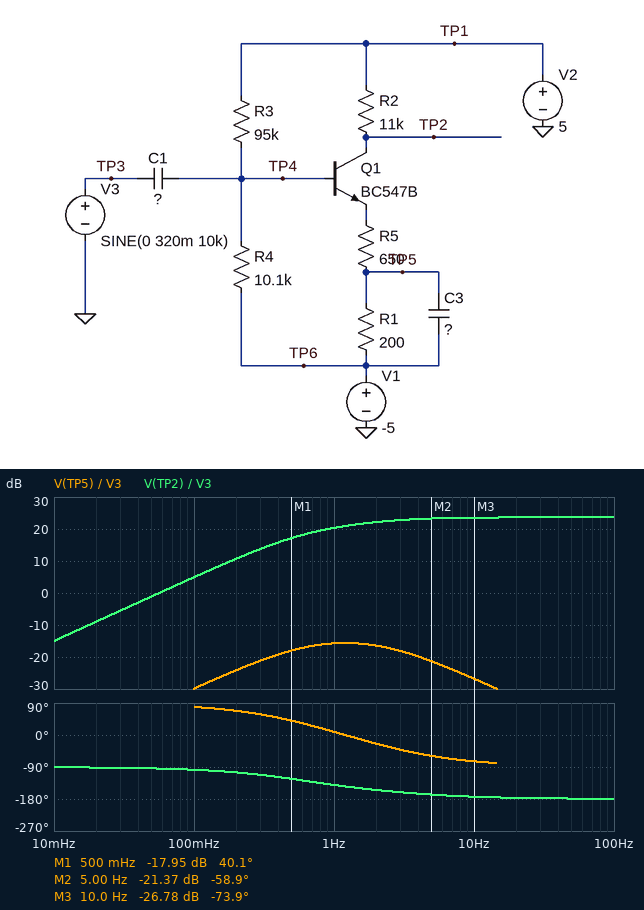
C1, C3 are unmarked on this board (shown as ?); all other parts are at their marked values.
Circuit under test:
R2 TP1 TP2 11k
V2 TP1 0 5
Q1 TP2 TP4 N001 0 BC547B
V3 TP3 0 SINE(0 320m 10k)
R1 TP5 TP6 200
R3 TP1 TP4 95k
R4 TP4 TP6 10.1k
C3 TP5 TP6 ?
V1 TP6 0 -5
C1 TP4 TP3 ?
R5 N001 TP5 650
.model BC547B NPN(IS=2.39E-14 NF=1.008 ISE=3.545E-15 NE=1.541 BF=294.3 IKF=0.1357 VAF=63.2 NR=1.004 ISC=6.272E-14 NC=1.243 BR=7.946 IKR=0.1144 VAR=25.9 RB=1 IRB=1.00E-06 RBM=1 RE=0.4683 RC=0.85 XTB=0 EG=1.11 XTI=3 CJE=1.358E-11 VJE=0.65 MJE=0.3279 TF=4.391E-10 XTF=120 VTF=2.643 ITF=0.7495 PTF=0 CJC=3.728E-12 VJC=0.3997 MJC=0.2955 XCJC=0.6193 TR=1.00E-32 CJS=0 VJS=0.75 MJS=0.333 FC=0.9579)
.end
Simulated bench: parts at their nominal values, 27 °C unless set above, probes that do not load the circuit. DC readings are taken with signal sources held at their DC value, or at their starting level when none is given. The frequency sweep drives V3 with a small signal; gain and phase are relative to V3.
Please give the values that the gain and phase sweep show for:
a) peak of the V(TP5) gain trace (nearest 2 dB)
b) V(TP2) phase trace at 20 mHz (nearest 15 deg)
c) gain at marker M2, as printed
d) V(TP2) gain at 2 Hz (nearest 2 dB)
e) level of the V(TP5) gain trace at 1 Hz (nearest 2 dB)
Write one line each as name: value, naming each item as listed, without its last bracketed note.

peak of the V(TP5) gain trace: -16 dB
V(TP2) phase trace at 20 mHz: -90 deg
gain at marker M2, as printed: -21.37 dB
V(TP2) gain at 2 Hz: 22 dB
level of the V(TP5) gain trace at 1 Hz: -16 dB
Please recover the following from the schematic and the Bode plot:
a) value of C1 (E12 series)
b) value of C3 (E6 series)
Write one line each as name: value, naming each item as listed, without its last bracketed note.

value of C1: 27 µF
value of C3: 470 µF
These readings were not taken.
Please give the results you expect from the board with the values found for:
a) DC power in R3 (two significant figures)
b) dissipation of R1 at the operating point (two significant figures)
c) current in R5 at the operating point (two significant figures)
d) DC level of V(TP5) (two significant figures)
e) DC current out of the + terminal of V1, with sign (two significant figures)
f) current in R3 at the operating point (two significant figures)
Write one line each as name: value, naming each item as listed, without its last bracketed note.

DC power in R3: 860 µW
dissipation of R1 at the operating point: 31 µW
current in R5 at the operating point: 400 µA
DC level of V(TP5): -4.9 V
DC current out of the + terminal of V1, with sign: -490 µA
current in R3 at the operating point: 95 µA
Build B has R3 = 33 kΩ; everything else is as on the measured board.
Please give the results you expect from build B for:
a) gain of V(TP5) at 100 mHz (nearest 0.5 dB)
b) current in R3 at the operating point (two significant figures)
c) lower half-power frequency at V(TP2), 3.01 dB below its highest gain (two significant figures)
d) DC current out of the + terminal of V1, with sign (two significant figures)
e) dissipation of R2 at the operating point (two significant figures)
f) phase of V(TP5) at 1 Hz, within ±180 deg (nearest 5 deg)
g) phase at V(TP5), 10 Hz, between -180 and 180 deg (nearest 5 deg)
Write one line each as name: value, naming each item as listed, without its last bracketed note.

gain of V(TP5) at 100 mHz: -51.0 dB
current in R3 at the operating point: 260 µA
lower half-power frequency at V(TP2), 3.01 dB below its highest gain: 8.9 Hz
DC current out of the + terminal of V1, with sign: -1.1 mA
dissipation of R2 at the operating point: 7.6 mW
phase of V(TP5) at 1 Hz, within ±180 deg: 55 deg
phase at V(TP5), 10 Hz, between -180 and 180 deg: -40 deg
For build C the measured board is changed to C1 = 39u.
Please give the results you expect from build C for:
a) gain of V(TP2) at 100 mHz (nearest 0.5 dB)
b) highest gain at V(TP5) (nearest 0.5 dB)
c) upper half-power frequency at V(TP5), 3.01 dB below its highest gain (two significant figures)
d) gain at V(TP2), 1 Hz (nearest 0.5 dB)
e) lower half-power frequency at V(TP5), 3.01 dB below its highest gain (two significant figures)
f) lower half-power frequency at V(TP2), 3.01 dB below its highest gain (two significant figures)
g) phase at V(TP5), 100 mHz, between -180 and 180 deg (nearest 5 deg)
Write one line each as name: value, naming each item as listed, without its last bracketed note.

gain of V(TP2) at 100 mHz: 8.0 dB
highest gain at V(TP5): -15.0 dB
upper half-power frequency at V(TP5), 3.01 dB below its highest gain: 3.0 Hz
gain at V(TP2), 1 Hz: 21.0 dB
lower half-power frequency at V(TP5), 3.01 dB below its highest gain: 340 mHz
lower half-power frequency at V(TP2), 3.01 dB below its highest gain: 820 mHz
phase at V(TP5), 100 mHz, between -180 and 180 deg: 75 deg
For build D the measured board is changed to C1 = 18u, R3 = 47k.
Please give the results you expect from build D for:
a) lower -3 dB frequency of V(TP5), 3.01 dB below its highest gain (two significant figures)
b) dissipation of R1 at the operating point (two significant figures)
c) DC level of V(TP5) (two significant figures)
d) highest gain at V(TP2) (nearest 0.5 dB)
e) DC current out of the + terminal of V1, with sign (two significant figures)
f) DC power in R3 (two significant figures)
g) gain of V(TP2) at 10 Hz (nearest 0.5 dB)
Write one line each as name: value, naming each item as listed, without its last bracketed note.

lower -3 dB frequency of V(TP5), 3.01 dB below its highest gain: 1.4 Hz
dissipation of R1 at the operating point: 160 µW
DC level of V(TP5): -4.8 V
highest gain at V(TP2): -13.5 dB
DC current out of the + terminal of V1, with sign: -1.0 mA
DC power in R3: 1.6 mW
gain of V(TP2) at 10 Hz: -17.0 dB
